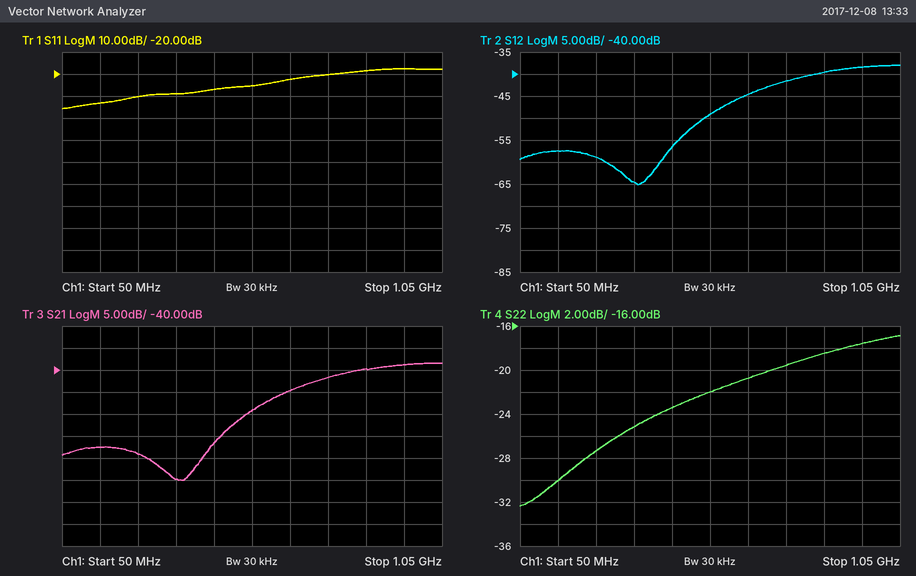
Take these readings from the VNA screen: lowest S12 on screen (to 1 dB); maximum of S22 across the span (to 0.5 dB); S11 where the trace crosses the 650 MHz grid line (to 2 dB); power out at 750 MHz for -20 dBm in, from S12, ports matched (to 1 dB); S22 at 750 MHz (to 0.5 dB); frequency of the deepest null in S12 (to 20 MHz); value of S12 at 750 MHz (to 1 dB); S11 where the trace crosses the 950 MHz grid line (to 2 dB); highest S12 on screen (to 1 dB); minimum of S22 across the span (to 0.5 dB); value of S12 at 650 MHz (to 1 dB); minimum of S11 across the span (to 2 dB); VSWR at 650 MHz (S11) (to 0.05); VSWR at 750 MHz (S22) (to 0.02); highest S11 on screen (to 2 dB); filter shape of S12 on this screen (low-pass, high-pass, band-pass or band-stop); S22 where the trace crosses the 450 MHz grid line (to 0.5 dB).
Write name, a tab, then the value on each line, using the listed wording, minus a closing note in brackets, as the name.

lowest S12 on screen	-65 dB
maximum of S22 across the span	-17.0 dB
S11 where the trace crosses the 650 MHz grid line	-22 dB
power out at 750 MHz for -20 dBm in, from S12, ports matched	-62 dBm
S22 at 750 MHz	-19.5 dB
frequency of the deepest null in S12	360 MHz
value of S12 at 750 MHz	-42 dB
S11 where the trace crosses the 950 MHz grid line	-18 dB
highest S12 on screen	-38 dB
minimum of S22 across the span	-32.5 dB
value of S12 at 650 MHz	-45 dB
minimum of S11 across the span	-36 dB
VSWR at 650 MHz (S11)	1.15
VSWR at 750 MHz (S22)	1.24
highest S11 on screen	-18 dB
filter shape of S12 on this screen	high-pass
S22 where the trace crosses the 450 MHz grid line	-23.5 dB
